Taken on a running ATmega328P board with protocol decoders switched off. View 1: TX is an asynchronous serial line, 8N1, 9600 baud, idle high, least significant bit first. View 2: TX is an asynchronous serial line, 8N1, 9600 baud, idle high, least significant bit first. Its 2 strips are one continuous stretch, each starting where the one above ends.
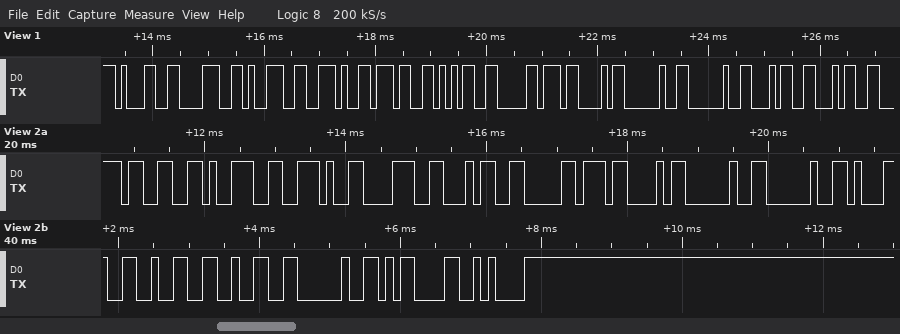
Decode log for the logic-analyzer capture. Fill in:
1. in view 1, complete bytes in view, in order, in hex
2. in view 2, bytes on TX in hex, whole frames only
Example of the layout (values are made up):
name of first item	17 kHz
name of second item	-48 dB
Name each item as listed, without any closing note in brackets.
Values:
in view 1, complete bytes in view, in order, in hex	31 38 39 2E 37 35 B0 43 20 20 34 34
in view 2, bytes on TX in hex, whole frames only	33 39 2E 38 34 B0 43 20 20 31 32 32 20 0D 0A
